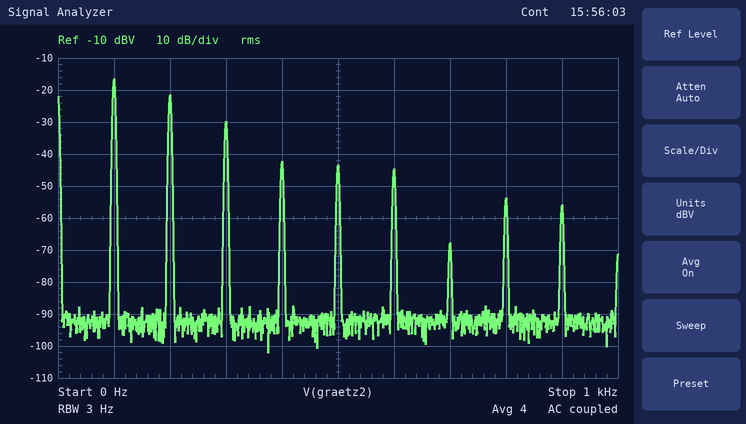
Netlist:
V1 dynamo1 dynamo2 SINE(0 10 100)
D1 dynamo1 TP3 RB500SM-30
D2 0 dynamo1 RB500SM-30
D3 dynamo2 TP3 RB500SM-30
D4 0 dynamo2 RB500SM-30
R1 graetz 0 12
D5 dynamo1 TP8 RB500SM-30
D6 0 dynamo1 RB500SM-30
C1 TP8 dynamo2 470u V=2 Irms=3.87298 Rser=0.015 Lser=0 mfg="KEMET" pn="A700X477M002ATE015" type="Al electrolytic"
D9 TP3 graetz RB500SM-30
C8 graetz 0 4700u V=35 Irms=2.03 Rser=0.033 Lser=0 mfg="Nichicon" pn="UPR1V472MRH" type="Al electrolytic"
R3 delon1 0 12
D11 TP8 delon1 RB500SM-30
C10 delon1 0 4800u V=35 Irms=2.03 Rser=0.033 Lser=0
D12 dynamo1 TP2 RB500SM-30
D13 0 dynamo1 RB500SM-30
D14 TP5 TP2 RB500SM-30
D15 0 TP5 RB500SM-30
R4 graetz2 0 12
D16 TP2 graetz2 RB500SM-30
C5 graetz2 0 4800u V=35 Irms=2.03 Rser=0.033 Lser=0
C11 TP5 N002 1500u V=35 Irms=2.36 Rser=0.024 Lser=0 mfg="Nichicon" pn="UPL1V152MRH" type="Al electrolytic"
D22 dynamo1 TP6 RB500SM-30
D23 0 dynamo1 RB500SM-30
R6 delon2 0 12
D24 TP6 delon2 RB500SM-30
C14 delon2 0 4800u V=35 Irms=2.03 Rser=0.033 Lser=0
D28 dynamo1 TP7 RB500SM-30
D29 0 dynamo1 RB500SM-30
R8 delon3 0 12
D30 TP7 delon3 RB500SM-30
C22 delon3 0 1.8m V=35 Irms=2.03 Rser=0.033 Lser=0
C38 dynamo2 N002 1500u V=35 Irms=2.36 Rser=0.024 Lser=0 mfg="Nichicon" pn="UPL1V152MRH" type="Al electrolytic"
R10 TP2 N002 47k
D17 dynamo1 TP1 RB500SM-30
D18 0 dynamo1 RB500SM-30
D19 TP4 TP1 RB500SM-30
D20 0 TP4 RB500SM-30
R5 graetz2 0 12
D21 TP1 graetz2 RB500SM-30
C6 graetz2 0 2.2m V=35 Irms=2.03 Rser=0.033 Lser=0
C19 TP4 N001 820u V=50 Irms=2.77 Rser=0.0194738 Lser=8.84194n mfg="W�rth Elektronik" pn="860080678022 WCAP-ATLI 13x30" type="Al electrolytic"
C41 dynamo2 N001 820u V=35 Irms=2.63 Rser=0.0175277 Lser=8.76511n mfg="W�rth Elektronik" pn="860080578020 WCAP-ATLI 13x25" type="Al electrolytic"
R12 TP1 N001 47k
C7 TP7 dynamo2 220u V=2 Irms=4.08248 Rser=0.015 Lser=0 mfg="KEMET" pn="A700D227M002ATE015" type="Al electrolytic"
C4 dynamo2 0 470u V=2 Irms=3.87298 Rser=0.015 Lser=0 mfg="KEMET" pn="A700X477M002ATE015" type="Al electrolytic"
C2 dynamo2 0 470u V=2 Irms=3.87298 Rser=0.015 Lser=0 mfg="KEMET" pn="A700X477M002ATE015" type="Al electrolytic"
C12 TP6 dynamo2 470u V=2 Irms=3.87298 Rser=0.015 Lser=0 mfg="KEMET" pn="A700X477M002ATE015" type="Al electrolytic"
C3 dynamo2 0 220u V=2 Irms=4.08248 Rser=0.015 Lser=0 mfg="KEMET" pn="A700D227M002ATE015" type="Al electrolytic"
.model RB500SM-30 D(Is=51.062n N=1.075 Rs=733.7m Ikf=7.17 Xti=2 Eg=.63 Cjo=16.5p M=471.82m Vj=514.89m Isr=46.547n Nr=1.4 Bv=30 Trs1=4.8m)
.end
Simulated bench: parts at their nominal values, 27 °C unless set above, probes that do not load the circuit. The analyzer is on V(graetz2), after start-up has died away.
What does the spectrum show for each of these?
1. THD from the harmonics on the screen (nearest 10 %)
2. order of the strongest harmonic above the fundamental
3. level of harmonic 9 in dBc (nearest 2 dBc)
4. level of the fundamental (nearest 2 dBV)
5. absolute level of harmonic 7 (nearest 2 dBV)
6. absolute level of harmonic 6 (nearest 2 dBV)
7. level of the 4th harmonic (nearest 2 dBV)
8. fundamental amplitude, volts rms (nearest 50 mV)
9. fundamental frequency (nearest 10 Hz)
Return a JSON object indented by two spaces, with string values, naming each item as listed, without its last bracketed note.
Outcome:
{
  "THD from the harmonics on the screen": "60 %",
  "order of the strongest harmonic above the fundamental": "2",
  "level of harmonic 9 in dBc": "-40 dBc",
  "level of the fundamental": "-16 dBV",
  "absolute level of harmonic 7": "-68 dBV",
  "absolute level of harmonic 6": "-44 dBV",
  "level of the 4th harmonic": "-42 dBV",
  "fundamental amplitude, volts rms": "150 mV",
  "fundamental frequency": "100 Hz"
}
